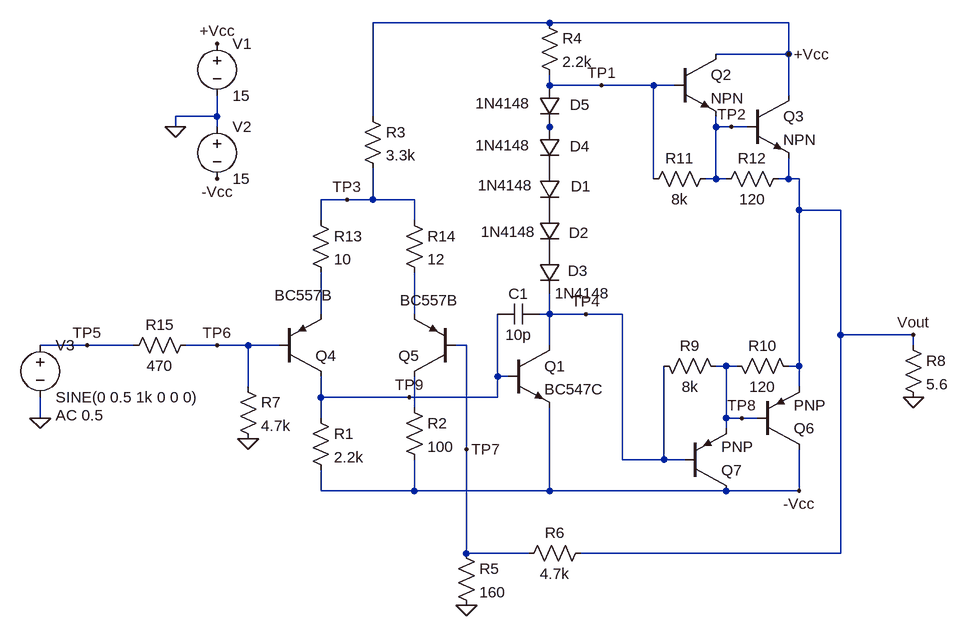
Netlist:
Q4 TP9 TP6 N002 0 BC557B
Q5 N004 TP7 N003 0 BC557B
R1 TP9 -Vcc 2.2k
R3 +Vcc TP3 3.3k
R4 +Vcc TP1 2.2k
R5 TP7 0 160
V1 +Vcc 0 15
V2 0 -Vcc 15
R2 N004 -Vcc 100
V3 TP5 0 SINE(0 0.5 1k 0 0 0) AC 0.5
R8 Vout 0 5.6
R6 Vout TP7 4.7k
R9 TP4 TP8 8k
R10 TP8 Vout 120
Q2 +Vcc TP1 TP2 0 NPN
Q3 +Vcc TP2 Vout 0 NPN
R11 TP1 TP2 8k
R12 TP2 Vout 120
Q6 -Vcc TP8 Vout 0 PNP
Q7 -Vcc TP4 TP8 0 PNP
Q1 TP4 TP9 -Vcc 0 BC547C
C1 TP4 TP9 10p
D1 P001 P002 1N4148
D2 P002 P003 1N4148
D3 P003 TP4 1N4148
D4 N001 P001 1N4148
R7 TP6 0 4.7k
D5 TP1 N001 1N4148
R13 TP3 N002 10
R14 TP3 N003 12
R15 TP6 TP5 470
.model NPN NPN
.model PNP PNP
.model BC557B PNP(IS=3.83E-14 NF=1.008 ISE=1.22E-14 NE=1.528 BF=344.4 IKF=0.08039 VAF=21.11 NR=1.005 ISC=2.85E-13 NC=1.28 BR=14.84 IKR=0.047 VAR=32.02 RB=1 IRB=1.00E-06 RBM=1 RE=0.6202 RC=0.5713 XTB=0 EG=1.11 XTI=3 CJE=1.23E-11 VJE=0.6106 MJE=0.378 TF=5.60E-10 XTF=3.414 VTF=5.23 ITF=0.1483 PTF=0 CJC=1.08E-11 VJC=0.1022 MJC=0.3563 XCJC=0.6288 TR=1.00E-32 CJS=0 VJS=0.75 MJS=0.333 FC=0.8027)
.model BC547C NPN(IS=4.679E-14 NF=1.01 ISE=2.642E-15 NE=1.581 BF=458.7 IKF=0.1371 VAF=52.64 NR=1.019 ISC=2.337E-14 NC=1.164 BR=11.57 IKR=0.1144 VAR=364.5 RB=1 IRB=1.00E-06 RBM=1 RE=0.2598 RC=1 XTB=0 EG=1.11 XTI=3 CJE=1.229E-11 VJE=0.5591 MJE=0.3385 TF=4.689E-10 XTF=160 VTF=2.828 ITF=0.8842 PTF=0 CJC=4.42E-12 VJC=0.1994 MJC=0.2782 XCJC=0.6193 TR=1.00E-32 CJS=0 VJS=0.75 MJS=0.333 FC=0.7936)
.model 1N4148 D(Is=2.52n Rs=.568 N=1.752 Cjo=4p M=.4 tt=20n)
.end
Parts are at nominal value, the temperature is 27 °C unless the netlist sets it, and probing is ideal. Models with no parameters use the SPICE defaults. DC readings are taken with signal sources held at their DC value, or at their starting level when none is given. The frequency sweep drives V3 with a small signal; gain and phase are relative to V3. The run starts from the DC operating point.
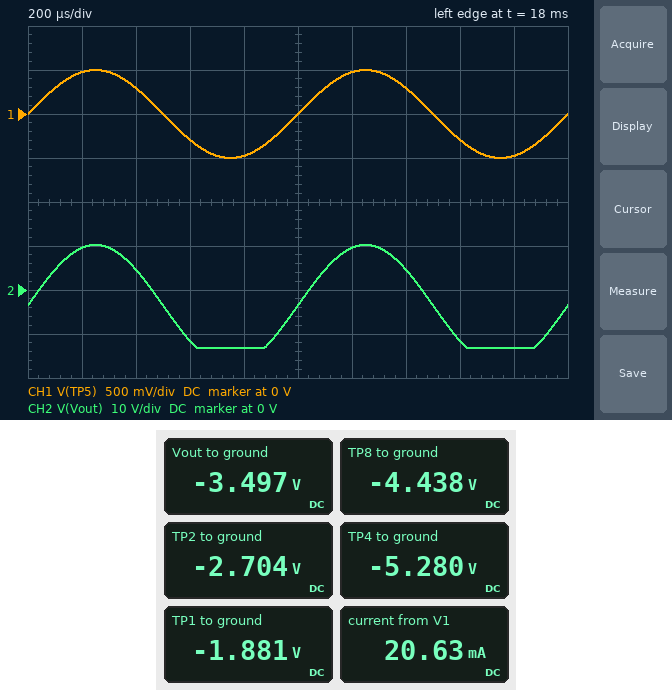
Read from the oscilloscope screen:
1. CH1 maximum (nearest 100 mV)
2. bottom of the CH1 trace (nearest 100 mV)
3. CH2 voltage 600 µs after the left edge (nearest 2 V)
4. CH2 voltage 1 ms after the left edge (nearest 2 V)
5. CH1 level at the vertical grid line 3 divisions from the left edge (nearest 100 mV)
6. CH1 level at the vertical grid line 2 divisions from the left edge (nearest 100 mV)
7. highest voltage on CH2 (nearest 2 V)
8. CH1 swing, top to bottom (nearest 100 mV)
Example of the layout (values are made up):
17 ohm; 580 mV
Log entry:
500 mV; -500 mV; -12 V; -4 V; -300 mV; 300 mV; 10 V; 1.0 V
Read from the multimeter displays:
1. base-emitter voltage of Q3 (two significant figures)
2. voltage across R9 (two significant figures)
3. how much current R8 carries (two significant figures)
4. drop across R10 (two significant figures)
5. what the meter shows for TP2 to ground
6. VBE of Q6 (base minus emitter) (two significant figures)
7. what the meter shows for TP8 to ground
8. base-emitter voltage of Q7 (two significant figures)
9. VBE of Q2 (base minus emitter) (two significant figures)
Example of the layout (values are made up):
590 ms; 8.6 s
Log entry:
790 mV; 840 mV; 620 mA; 940 mV; -2.704 V; -940 mV; -4.438 V; -840 mV; 820 mV
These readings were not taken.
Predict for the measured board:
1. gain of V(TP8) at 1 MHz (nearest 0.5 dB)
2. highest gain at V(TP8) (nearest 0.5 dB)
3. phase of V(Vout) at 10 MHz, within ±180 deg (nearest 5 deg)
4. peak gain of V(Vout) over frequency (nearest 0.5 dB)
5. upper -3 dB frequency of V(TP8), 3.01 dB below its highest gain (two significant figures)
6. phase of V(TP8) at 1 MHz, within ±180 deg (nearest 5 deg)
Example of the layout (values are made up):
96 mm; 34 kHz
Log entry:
29.0 dB; 29.0 dB; -120 deg; 29.0 dB; 5.4 MHz; -15 deg
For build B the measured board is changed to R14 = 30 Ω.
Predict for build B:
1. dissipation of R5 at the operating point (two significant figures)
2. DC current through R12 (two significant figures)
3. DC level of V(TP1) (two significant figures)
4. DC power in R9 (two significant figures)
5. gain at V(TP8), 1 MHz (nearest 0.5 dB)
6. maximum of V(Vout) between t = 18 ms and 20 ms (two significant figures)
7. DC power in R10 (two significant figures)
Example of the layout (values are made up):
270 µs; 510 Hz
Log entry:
220 µW; 6.7 mA; -4.1 V; 90 µW; 28.5 dB; 8.1 V; 7.6 mW
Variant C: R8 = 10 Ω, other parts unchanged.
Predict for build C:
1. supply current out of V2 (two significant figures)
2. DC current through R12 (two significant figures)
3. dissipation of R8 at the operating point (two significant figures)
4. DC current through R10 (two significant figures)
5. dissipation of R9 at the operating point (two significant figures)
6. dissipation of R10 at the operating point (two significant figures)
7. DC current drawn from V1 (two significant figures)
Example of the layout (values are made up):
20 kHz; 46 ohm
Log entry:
370 mA; 6.8 mA; 1.2 W; 7.7 mA; 87 µW; 7.1 mW; 23 mA
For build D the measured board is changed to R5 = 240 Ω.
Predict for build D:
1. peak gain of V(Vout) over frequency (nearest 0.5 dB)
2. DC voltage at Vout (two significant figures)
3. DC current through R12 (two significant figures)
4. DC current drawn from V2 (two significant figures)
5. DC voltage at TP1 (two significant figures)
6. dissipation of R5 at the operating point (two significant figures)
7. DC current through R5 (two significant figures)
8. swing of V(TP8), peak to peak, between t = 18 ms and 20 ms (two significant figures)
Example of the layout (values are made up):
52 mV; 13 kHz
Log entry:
25.5 dB; -2.4 V; 6.6 mA; 450 mA; -770 mV; 54 µW; 480 µA; 19 V
